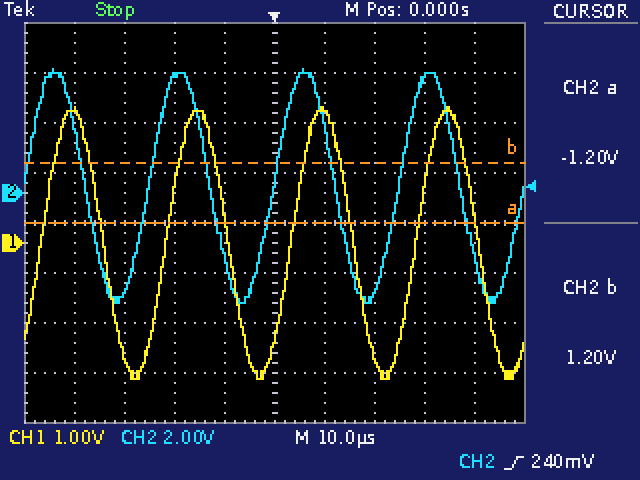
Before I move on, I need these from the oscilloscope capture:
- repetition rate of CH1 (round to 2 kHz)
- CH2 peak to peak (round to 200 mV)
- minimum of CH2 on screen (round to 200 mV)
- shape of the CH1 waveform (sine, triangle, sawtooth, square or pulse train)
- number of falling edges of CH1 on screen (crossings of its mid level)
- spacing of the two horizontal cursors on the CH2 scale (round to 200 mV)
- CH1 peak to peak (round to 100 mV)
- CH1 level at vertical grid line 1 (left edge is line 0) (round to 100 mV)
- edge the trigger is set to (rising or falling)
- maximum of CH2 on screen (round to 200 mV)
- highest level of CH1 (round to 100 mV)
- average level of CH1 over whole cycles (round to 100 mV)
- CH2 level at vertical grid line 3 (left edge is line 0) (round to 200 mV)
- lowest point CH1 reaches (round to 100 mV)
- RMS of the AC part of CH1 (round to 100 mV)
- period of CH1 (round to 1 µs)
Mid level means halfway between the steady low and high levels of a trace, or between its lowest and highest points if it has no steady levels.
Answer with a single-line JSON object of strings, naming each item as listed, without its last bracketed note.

{"repetition rate of CH1": "40 kHz", "CH2 peak to peak": "9.4 V", "minimum of CH2 on screen": "-4.4 V", "shape of the CH1 waveform": "sine", "number of falling edges of CH1 on screen": "4", "spacing of the two horizontal cursors on the CH2 scale": "2.4 V", "CH1 peak to peak": "5.4 V", "CH1 level at vertical grid line 1 (left edge is line 0)": "2.6 V", "edge the trigger is set to": "rising", "maximum of CH2 on screen": "5.0 V", "highest level of CH1": "2.7 V", "average level of CH1 over whole cycles": "0.0 V", "CH2 level at vertical grid line 3 (left edge is line 0)": "4.6 V", "lowest point CH1 reaches": "-2.7 V", "RMS of the AC part of CH1": "1.9 V", "period of CH1": "25 µs"}
